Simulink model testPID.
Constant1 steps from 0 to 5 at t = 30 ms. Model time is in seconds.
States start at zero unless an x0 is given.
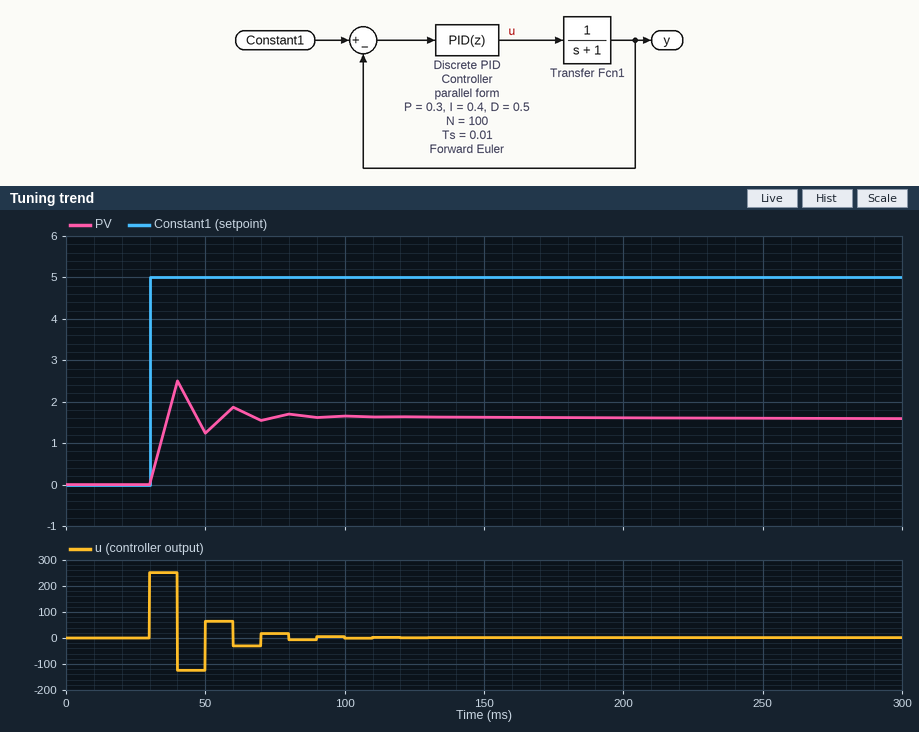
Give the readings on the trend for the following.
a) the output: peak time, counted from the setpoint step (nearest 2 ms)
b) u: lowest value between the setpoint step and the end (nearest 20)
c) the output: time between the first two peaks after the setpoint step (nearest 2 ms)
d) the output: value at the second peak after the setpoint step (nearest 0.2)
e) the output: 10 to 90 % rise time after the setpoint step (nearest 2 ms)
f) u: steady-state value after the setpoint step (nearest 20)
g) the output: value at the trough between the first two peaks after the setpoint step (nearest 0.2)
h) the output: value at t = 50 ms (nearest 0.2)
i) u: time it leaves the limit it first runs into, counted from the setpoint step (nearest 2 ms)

10 ms
-120
20 ms
1.8
6 ms
0
1.2
1.2
10 ms
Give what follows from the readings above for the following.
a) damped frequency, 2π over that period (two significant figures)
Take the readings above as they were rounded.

0.31 rad/ms
